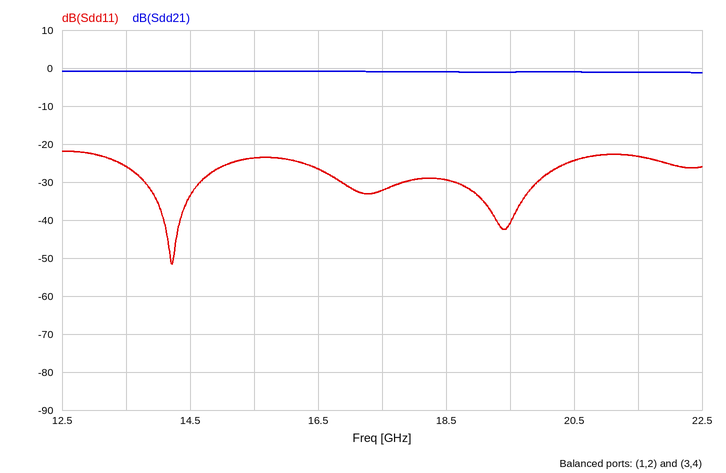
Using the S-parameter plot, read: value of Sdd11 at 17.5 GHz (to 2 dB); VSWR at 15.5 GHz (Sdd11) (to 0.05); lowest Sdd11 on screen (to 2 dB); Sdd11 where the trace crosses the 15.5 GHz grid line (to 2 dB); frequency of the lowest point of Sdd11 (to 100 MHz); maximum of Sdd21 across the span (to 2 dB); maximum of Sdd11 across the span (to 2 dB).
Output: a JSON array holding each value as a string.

["-32 dB", "1.15", "-52 dB", "-24 dB", "14.2 GHz", "0 dB", "-22 dB"]
